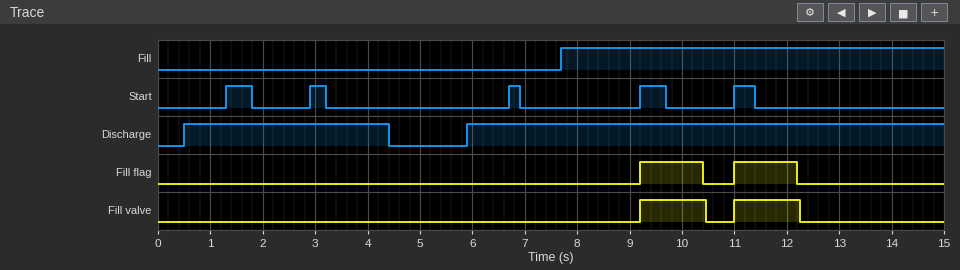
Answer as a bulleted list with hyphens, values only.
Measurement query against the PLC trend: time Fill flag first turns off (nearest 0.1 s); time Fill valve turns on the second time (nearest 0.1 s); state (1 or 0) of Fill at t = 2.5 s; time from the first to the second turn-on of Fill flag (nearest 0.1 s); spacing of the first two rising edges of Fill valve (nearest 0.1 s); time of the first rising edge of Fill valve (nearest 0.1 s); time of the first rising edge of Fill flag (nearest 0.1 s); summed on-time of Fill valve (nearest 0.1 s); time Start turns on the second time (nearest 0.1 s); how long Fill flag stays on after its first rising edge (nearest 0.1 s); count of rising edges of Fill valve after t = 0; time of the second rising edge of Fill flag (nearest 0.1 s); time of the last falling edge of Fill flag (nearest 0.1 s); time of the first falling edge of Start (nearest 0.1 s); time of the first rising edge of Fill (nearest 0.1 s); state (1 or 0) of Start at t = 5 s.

- 10.4 s
- 11.0 s
- 0
- 1.8 s
- 1.8 s
- 9.2 s
- 9.2 s
- 2.5 s
- 2.9 s
- 1.2 s
- 2
- 11.0 s
- 12.2 s
- 1.8 s
- 7.7 s
- 0
